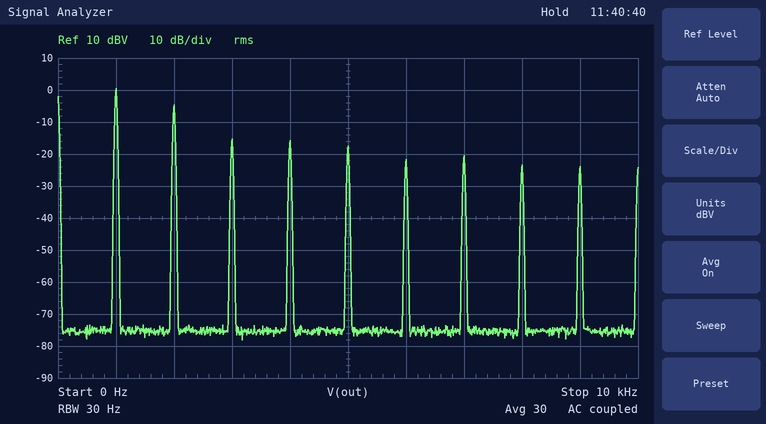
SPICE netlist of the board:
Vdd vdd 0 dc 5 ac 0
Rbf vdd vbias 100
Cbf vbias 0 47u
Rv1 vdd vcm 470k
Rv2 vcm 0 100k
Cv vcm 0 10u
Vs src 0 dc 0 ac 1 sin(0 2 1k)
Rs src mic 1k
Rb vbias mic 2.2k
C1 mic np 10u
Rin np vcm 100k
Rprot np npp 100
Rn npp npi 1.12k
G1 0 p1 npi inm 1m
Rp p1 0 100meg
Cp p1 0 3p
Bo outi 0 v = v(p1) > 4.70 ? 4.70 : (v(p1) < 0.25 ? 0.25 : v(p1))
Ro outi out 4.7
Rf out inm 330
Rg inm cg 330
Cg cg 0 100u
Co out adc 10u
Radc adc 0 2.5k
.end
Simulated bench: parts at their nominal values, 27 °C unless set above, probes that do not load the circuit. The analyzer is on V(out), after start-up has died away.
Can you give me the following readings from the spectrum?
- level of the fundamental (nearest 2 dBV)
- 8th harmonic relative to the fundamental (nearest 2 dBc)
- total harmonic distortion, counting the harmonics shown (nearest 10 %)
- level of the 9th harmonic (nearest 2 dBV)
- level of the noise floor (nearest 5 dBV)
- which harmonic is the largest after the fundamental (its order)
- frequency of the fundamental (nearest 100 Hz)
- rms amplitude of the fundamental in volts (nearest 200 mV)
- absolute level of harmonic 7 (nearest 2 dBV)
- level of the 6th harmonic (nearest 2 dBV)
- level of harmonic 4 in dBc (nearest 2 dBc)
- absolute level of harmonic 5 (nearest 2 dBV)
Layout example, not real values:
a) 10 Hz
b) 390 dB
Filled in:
a) 0 dBV
b) -24 dBc
c) 60 %
d) -24 dBV
e) -75 dBV
f) 2
g) 1.0 kHz
h) 1.0 V
i) -20 dBV
j) -22 dBV
k) -16 dBc
l) -18 dBV
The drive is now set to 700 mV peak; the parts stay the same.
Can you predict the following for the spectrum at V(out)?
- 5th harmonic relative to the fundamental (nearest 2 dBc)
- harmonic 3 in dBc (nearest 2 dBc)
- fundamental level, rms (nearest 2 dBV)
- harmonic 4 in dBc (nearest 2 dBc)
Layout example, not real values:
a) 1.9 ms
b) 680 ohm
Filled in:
a) -26 dBc
b) -18 dBc
c) -4 dBV
d) -26 dBc
